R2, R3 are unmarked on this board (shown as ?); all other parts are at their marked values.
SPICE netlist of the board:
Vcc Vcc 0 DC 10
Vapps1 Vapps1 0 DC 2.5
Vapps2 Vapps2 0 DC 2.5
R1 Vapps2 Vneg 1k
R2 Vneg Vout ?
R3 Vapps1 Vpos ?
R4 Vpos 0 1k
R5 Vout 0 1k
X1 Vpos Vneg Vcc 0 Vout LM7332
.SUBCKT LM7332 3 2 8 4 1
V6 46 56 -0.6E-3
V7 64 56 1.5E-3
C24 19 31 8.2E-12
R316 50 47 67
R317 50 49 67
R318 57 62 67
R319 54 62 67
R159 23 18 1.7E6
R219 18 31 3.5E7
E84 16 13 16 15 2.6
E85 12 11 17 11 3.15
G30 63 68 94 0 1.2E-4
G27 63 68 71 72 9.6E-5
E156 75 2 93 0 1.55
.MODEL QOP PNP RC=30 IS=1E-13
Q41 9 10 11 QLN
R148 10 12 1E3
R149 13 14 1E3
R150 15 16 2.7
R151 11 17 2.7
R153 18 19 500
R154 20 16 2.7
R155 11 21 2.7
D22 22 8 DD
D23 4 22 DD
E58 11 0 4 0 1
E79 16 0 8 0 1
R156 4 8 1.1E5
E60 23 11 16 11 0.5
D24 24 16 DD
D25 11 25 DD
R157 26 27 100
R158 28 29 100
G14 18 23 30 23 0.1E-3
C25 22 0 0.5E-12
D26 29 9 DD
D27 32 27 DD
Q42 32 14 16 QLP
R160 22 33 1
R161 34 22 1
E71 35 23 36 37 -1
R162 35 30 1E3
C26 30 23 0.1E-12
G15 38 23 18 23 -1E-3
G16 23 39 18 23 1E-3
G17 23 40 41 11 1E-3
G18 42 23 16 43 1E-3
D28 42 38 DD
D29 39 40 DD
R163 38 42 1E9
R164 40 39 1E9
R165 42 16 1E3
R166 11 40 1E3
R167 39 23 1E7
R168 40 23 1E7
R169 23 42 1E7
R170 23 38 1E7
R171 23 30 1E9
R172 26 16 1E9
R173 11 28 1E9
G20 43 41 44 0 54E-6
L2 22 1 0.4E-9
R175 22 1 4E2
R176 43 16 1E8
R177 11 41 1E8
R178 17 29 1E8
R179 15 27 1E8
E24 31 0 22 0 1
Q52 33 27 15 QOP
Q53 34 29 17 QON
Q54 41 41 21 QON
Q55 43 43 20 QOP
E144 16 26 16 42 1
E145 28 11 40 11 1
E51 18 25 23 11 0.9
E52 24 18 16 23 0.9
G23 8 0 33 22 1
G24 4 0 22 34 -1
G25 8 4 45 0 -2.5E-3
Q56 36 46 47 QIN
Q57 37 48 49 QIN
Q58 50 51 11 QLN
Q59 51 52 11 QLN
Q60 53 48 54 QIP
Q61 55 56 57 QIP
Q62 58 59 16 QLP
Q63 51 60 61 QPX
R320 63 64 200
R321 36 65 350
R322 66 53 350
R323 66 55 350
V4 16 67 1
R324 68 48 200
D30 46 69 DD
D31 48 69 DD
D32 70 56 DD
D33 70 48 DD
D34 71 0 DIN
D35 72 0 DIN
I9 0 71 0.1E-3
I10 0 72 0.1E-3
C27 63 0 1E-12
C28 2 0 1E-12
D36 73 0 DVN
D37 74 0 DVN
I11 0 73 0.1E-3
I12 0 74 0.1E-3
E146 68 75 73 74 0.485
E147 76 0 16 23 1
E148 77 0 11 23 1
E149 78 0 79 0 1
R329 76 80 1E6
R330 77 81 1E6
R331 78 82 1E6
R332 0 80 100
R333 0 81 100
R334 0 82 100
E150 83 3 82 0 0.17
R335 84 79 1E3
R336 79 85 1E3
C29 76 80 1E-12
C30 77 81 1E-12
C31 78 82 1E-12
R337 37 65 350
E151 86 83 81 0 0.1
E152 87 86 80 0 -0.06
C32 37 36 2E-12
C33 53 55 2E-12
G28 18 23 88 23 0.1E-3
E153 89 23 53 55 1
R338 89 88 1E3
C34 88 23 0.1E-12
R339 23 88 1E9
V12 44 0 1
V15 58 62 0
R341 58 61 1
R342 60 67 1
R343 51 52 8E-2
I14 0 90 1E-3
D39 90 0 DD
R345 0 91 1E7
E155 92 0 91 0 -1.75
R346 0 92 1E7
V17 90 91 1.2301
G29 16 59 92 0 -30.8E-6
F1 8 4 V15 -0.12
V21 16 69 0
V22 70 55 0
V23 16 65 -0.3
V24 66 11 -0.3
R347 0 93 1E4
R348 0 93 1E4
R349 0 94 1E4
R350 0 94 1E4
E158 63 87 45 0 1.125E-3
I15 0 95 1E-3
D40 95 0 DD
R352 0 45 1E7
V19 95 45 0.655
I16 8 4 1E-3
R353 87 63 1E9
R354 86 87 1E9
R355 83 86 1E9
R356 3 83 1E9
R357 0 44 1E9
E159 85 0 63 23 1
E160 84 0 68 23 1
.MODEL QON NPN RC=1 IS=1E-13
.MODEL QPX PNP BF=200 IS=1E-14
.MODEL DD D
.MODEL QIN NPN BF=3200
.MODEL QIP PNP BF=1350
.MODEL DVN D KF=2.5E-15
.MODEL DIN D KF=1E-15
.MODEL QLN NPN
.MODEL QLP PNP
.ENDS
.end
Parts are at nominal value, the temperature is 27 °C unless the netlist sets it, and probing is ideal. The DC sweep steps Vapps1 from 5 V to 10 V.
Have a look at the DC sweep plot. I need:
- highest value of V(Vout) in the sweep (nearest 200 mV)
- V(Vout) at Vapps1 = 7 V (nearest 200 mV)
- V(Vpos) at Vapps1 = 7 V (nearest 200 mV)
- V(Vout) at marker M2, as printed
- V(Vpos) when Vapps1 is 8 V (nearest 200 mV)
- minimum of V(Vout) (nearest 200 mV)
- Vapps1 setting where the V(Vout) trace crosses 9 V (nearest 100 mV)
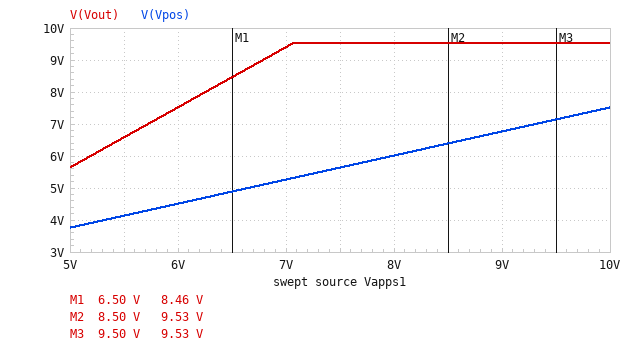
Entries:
9.6 V
9.4 V
5.2 V
9.53 V
6.0 V
5.6 V
6.8 V
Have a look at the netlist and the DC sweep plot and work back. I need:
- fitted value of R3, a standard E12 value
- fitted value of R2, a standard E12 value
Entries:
330 Ω
1.5 kΩ
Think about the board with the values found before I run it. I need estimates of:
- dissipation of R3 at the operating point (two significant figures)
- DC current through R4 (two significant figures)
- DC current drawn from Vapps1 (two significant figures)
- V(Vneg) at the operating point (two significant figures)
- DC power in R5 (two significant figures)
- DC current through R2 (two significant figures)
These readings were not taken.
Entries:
1.2 mW
1.9 mA
1.9 mA
1.9 V
890 µW
620 µA
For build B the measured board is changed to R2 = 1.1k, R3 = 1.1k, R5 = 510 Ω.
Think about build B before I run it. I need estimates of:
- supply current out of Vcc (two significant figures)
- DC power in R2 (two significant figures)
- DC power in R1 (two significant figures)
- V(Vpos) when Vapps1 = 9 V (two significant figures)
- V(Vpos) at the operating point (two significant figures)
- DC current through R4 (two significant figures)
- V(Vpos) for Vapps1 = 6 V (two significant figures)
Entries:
750 µA
1.5 mW
1.4 mW
4.3 V
1.2 V
1.2 mA
2.9 V
